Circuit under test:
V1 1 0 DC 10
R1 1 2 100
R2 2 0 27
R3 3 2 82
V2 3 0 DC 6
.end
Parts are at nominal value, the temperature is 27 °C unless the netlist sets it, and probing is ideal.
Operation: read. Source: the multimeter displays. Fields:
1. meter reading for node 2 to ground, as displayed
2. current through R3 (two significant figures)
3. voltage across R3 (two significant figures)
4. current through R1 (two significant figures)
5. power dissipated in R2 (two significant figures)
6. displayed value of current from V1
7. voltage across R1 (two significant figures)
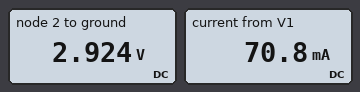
2.924 V
38 mA
3.1 V
71 mA
320 mW
70.8 mA
7.1 V
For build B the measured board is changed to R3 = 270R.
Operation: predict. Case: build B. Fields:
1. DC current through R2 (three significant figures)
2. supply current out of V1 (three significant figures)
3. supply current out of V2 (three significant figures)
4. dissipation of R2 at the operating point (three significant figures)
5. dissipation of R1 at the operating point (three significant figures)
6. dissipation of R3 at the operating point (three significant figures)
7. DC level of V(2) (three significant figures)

89.2 mA
75.9 mA
13.3 mA
215 mW
576 mW
47.8 mW
2.41 V
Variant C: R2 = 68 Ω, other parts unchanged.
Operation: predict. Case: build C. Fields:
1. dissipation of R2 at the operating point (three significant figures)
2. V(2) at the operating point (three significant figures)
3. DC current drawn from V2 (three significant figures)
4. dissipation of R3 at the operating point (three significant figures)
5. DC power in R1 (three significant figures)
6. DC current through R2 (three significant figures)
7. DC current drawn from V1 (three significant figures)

324 mW
4.69 V
15.9 mA
20.8 mW
282 mW
69.0 mA
53.1 mA
